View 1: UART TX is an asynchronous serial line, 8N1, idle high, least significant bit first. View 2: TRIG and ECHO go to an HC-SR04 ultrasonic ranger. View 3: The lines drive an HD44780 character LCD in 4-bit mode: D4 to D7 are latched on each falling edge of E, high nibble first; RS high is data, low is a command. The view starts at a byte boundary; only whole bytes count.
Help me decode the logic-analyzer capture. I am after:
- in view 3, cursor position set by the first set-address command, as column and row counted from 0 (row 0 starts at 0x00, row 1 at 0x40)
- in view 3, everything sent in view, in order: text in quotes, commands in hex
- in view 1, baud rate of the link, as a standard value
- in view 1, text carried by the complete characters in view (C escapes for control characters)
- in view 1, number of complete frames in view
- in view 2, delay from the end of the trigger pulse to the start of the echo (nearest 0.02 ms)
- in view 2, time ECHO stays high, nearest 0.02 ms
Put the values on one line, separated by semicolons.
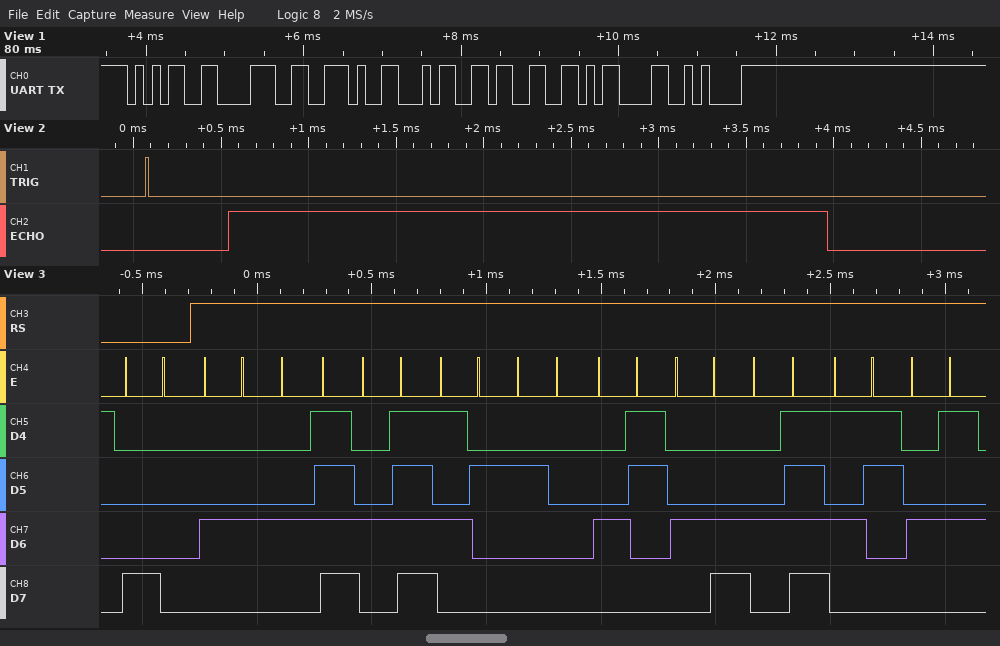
column 0, row 0; 0x80 "DOOR CLOSE"; 9600 baud; "58.43\r\n"; 7; 0.46 ms; 3.42 ms
